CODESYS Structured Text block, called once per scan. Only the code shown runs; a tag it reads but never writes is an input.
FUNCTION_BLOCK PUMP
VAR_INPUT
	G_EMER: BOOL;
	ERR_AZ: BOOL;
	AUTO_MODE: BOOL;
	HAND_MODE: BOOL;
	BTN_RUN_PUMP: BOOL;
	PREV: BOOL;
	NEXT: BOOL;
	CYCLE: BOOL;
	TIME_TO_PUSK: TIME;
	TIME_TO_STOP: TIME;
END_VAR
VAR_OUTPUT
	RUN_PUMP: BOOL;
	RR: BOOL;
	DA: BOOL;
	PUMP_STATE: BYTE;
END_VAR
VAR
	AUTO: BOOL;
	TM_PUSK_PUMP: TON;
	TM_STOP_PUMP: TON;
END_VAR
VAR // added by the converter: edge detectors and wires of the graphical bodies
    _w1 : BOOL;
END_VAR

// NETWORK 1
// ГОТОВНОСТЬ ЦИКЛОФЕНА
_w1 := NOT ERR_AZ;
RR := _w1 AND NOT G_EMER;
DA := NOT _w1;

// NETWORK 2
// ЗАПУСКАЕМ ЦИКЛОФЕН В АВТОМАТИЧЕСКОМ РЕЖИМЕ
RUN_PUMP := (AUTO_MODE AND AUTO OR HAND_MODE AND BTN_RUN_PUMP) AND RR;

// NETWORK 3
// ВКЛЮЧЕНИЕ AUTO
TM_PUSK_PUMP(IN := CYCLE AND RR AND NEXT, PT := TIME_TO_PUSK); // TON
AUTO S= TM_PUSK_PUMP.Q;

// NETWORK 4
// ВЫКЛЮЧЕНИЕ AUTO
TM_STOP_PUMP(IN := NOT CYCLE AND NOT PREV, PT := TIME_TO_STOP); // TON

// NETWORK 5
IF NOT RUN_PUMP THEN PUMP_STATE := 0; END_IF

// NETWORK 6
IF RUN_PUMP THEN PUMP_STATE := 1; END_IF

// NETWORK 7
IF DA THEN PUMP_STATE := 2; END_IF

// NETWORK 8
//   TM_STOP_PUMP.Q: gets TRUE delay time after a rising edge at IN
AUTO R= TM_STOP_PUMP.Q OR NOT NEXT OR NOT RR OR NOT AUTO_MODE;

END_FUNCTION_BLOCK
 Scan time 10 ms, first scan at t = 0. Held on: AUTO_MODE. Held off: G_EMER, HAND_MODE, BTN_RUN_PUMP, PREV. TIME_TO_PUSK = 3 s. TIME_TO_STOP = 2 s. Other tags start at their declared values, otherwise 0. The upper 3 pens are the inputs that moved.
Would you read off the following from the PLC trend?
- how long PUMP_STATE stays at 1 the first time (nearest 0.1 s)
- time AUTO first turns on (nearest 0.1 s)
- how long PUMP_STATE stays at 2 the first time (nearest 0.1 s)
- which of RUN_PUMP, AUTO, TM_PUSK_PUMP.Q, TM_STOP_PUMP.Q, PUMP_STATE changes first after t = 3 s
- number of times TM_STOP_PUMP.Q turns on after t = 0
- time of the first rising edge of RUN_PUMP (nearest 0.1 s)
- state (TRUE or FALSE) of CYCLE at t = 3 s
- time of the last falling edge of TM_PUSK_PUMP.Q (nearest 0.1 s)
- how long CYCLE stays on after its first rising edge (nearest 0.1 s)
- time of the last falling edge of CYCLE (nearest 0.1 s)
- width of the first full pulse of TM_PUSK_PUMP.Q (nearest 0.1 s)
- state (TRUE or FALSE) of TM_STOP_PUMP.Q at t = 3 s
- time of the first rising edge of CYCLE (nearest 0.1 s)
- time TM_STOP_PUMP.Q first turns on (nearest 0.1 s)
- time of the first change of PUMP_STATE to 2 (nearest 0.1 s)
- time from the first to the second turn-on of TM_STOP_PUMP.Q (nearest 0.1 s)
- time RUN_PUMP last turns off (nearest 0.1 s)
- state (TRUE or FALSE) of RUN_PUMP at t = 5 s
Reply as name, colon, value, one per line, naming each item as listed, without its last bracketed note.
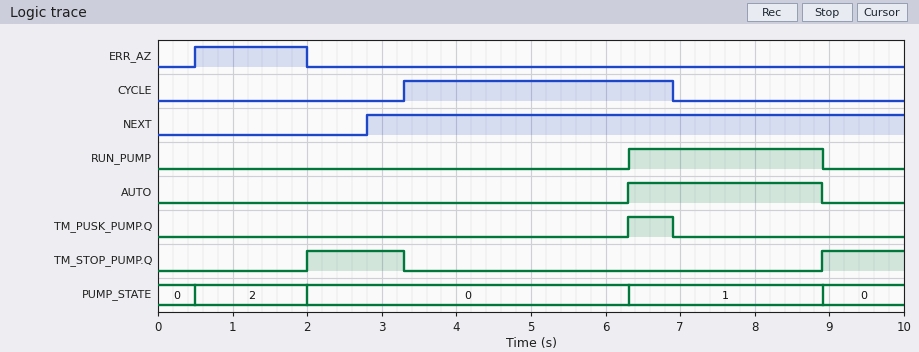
how long PUMP_STATE stays at 1 the first time: 2.6 s
time AUTO first turns on: 6.3 s
how long PUMP_STATE stays at 2 the first time: 1.5 s
which of RUN_PUMP, AUTO, TM_PUSK_PUMP.Q, TM_STOP_PUMP.Q, PUMP_STATE changes first after t = 3 s: TM_STOP_PUMP.Q
number of times TM_STOP_PUMP.Q turns on after t = 0: 2
time of the first rising edge of RUN_PUMP: 6.3 s
state (TRUE or FALSE) of CYCLE at t = 3 s: FALSE
time of the last falling edge of TM_PUSK_PUMP.Q: 6.9 s
how long CYCLE stays on after its first rising edge: 3.6 s
time of the last falling edge of CYCLE: 6.9 s
width of the first full pulse of TM_PUSK_PUMP.Q: 0.6 s
state (TRUE or FALSE) of TM_STOP_PUMP.Q at t = 3 s: TRUE
time of the first rising edge of CYCLE: 3.3 s
time TM_STOP_PUMP.Q first turns on: 2.0 s
time of the first change of PUMP_STATE to 2: 0.5 s
time from the first to the second turn-on of TM_STOP_PUMP.Q: 6.9 s
time RUN_PUMP last turns off: 8.9 s
state (TRUE or FALSE) of RUN_PUMP at t = 5 s: FALSE
